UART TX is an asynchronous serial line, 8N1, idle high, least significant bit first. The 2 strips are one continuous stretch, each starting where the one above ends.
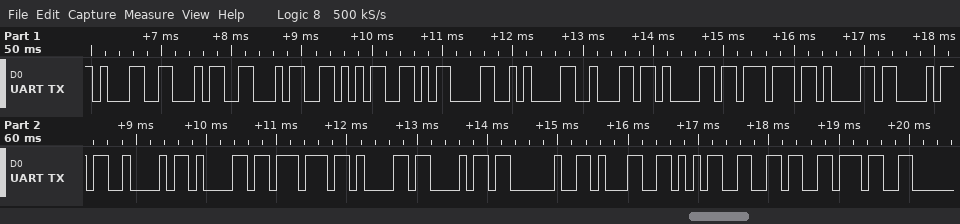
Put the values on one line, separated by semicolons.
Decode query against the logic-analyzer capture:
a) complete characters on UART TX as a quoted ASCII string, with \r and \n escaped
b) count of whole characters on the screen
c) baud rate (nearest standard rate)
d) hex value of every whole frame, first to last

"1445\r\nbawahBawah 1567"; 21; 9600 baud; 31 34 34 35 0D 0A 62 61 77 61 68 42 61 77 61 68 20 31 35 36 37
